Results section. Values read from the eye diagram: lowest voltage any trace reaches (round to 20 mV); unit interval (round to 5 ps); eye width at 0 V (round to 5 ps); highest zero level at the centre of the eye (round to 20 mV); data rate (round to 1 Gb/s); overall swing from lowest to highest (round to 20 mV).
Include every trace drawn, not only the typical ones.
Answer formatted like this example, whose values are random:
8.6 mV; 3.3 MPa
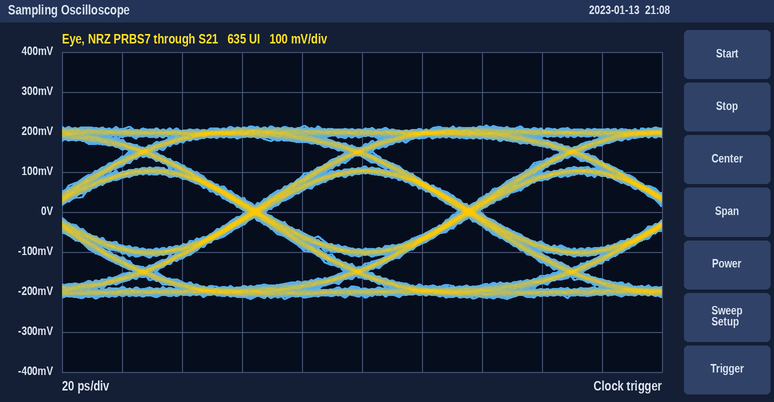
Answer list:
-220 mV; 70 ps; 65 ps; -100 mV; 14 Gb/s; 440 mV
